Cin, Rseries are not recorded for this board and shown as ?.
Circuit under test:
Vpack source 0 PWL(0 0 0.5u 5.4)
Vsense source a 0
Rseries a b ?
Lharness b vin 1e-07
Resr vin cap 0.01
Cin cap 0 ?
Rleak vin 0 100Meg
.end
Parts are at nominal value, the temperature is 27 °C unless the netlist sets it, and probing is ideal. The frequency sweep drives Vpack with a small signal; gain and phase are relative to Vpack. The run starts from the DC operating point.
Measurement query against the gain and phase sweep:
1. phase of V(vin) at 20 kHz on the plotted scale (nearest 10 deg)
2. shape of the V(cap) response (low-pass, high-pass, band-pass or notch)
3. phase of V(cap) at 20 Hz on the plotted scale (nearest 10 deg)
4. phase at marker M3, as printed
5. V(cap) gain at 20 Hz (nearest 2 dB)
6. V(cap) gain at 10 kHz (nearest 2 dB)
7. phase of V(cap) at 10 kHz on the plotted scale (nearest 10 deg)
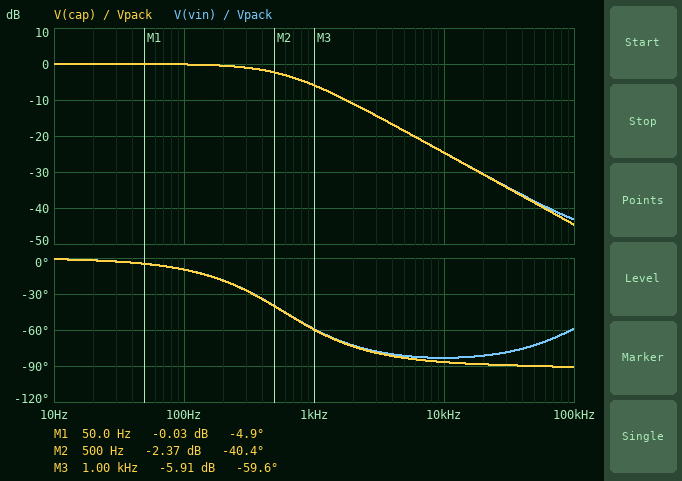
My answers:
-80 deg
low-pass
0 deg
-59.6 deg
0 dB
-24 dB
-90 deg
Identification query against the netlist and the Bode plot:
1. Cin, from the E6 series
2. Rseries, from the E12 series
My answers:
100 µF
2.7 Ω
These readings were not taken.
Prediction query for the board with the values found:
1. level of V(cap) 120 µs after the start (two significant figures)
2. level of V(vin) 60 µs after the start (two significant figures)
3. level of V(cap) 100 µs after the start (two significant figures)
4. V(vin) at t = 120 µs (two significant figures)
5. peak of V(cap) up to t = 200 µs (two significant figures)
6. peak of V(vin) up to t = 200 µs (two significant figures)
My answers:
1.9 V
1.1 V
1.7 V
1.9 V
2.8 V
2.8 V
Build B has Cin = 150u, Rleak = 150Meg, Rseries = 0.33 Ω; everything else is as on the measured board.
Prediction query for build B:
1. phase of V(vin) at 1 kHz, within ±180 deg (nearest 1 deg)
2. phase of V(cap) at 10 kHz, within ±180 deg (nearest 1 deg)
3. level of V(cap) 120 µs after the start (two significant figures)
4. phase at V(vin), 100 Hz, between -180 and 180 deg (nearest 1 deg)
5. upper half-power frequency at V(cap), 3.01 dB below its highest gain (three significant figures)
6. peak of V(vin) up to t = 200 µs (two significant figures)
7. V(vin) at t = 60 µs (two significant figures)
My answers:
-17 deg
-74 deg
4.9 V
-2 deg
3.14 kHz
5.3 V
3.8 V
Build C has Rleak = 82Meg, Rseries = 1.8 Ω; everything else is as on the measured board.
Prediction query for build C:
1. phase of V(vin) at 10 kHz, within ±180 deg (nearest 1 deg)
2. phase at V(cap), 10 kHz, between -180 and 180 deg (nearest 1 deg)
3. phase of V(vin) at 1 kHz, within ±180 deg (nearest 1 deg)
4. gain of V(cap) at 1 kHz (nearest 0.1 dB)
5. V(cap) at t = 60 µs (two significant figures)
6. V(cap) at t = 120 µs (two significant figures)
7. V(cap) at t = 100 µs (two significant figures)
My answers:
-82 deg
-85 deg
-48 deg
-3.6 dB
1.5 V
2.6 V
2.3 V
